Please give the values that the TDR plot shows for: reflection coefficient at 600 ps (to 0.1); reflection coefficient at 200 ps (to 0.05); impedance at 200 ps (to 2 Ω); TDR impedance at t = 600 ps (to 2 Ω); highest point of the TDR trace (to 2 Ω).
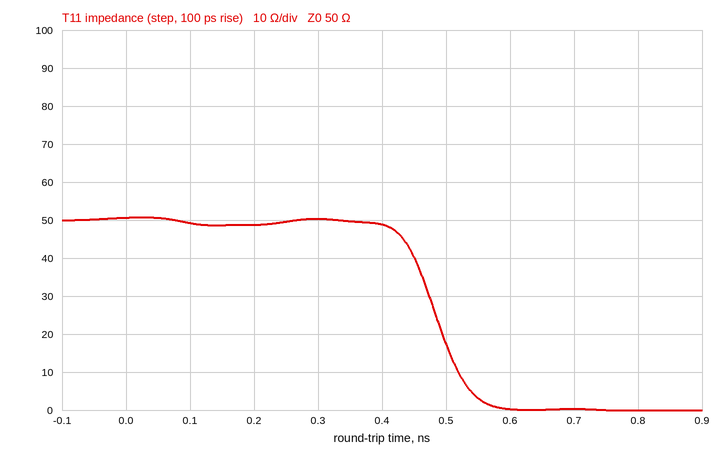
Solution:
-1.0
0.00
48 Ω
0 Ω
50 Ω
